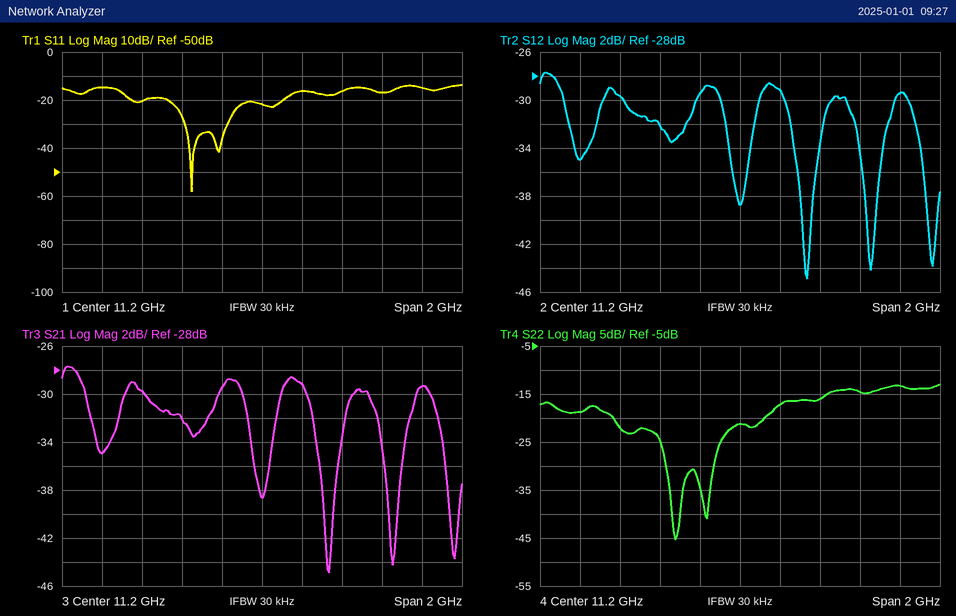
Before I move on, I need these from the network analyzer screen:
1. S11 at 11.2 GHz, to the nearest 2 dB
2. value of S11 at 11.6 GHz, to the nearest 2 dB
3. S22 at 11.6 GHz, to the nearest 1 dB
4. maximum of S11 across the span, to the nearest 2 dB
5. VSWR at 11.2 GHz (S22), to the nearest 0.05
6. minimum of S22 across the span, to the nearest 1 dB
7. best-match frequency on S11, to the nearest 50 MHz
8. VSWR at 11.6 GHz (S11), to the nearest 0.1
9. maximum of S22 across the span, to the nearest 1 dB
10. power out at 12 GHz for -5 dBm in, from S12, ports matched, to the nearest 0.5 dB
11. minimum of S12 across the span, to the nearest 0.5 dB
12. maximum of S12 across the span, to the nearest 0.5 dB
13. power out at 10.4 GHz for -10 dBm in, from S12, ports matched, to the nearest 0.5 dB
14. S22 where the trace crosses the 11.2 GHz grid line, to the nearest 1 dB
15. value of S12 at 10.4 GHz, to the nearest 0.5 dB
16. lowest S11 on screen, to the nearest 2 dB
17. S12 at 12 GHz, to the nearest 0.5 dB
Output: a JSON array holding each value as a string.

["-22 dB", "-16 dB", "-16 dB", "-14 dB", "1.20", "-45 dB", "10.85 GHz", "1.4", "-13 dB", "-34.5 dBm", "-45.0 dB", "-27.5 dB", "-45.0 dBm", "-21 dB", "-35.0 dB", "-58 dB", "-29.5 dB"]
